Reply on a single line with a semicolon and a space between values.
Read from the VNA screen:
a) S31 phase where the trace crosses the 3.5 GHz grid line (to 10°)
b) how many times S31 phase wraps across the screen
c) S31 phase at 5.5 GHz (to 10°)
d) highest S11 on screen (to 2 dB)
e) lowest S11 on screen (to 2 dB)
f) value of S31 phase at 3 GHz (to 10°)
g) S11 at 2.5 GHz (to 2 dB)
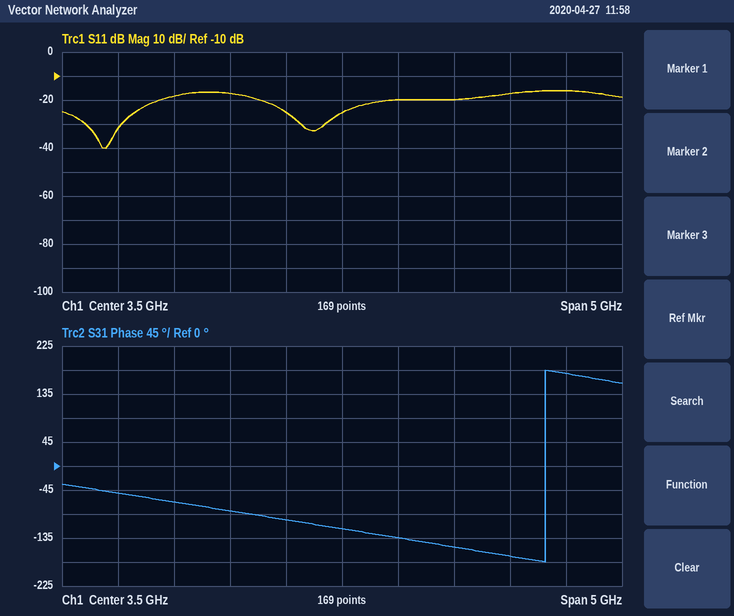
-120°; 1; 170°; -16 dB; -40 dB; -100°; -18 dB
